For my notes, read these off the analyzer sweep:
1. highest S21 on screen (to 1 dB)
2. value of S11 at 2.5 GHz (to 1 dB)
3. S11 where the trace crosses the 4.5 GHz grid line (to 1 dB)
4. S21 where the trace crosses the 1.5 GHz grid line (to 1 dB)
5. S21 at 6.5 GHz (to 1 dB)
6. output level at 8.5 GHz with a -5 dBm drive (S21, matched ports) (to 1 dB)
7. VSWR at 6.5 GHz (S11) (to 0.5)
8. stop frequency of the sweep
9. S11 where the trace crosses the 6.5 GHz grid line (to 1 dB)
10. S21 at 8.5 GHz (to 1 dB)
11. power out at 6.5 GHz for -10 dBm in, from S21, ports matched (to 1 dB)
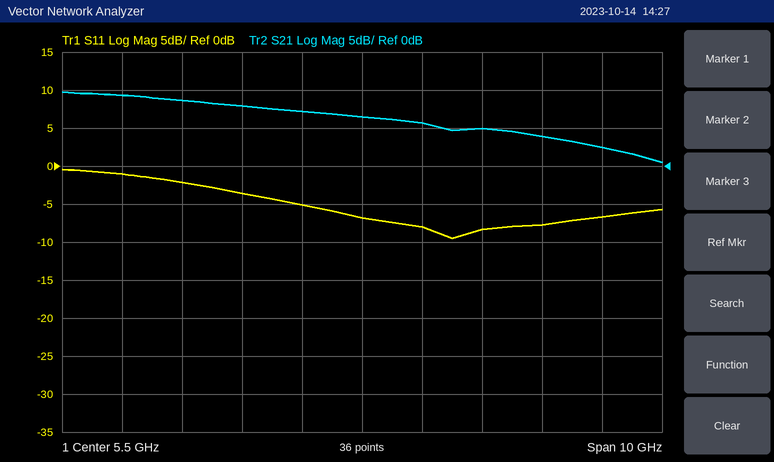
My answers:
10 dB
-2 dB
-5 dB
9 dB
6 dB
-1 dBm
2.5
10.5 GHz
-8 dB
4 dB
-4 dBm
